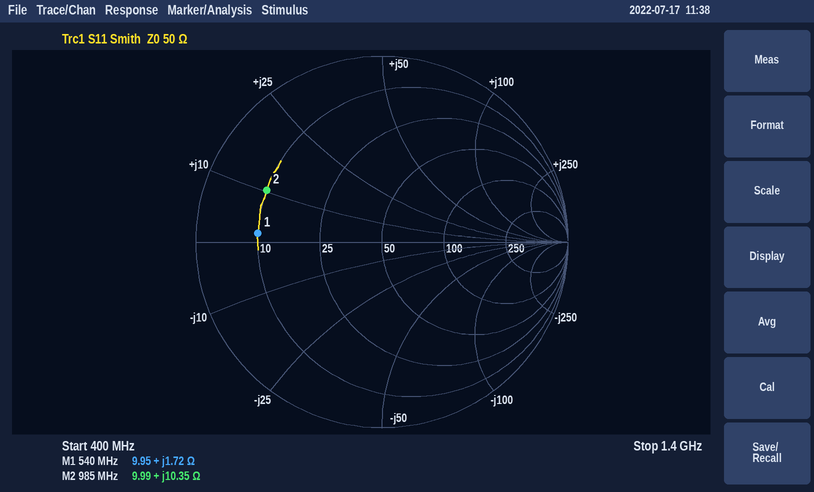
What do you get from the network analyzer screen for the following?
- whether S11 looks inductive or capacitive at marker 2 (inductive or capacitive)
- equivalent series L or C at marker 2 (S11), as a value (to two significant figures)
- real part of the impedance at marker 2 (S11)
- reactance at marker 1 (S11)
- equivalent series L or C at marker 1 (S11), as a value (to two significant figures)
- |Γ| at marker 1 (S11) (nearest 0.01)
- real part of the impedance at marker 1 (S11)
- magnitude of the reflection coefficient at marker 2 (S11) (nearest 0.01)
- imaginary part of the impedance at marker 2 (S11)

inductive
1.7 nH
9.99 Ω
+1.72 Ω
510 pH
0.67
9.95 Ω
0.68
+10.35 Ω
